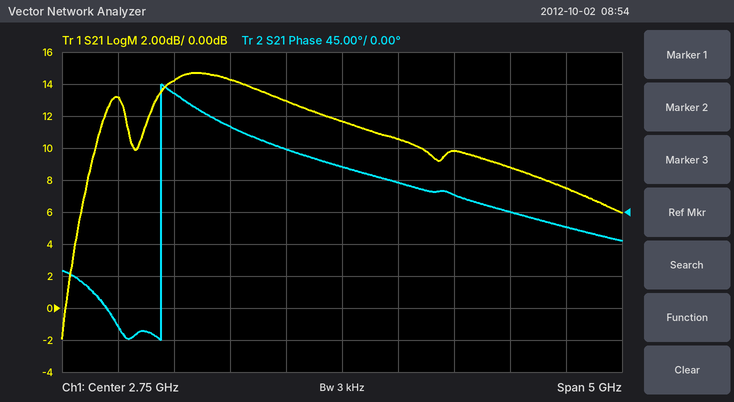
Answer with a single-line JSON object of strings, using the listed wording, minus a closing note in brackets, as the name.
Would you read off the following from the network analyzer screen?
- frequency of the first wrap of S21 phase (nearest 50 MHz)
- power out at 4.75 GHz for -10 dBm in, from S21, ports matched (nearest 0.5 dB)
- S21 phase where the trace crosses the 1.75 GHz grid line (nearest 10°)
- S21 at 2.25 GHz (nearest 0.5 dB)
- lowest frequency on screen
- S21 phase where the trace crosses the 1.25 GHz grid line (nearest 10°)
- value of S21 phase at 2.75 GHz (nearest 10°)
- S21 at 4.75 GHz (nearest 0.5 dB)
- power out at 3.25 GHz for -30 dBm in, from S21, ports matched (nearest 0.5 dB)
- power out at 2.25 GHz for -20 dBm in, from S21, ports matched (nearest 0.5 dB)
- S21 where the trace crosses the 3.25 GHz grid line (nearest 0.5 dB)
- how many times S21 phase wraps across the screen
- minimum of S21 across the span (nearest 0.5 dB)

{"frequency of the first wrap of S21 phase": "1.15 GHz", "power out at 4.75 GHz for -10 dBm in, from S21, ports matched": "-2.5 dBm", "S21 phase where the trace crosses the 1.75 GHz grid line": "120°", "S21 at 2.25 GHz": "13.0 dB", "lowest frequency on screen": "250 MHz", "S21 phase where the trace crosses the 1.25 GHz grid line": "170°", "value of S21 phase at 2.75 GHz": "60°", "S21 at 4.75 GHz": "7.5 dB", "power out at 3.25 GHz for -30 dBm in, from S21, ports matched": "-19.5 dBm", "power out at 2.25 GHz for -20 dBm in, from S21, ports matched": "-7.0 dBm", "S21 where the trace crosses the 3.25 GHz grid line": "10.5 dB", "how many times S21 phase wraps across the screen": "1", "minimum of S21 across the span": "-2.0 dB"}
